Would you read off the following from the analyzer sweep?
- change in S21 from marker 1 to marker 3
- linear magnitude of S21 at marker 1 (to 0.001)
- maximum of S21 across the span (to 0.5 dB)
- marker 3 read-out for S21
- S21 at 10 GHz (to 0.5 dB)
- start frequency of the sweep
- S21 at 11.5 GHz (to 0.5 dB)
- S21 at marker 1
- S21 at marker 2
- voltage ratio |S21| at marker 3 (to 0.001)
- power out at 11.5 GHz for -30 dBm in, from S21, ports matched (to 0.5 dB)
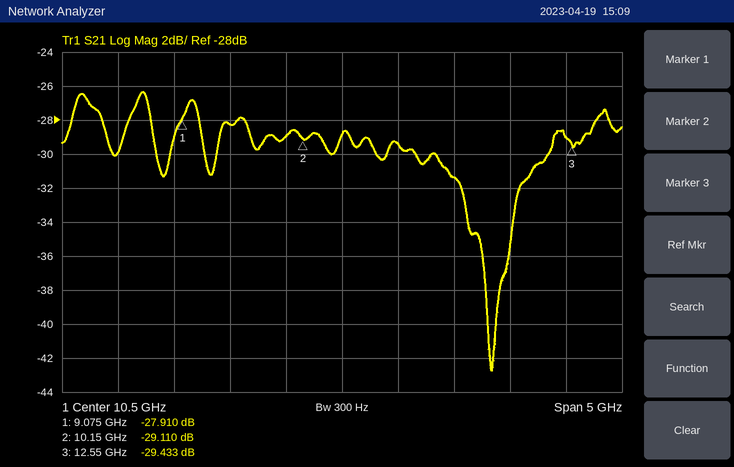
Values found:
-1.523 dB
0.040
-26.5 dB
-29.433 dB
-29.0 dB
8 GHz
-31.5 dB
-27.910 dB
-29.110 dB
0.034
-61.5 dBm
